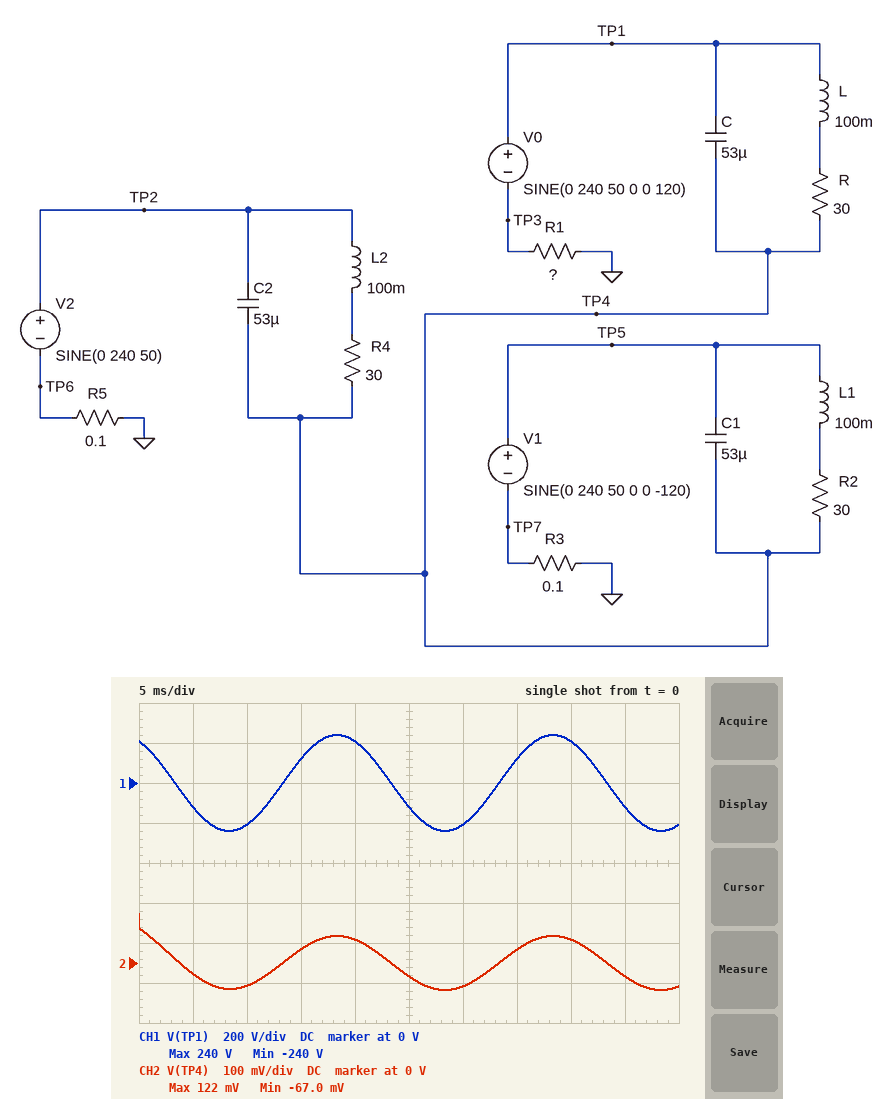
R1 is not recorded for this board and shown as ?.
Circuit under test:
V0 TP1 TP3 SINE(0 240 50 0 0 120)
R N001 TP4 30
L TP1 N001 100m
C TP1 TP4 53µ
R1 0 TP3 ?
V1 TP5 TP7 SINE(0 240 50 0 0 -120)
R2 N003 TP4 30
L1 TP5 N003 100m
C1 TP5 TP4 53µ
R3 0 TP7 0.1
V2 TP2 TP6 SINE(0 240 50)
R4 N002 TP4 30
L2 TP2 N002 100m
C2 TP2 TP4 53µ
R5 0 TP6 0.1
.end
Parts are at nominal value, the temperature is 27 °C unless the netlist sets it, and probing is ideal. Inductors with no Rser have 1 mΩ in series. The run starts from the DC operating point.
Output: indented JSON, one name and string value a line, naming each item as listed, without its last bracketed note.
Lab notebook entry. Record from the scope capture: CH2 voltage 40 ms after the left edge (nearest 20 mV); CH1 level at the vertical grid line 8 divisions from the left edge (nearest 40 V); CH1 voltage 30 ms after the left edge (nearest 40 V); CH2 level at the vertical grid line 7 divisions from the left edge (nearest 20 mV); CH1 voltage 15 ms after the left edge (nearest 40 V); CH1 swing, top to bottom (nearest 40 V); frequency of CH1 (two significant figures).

{
  "CH2 voltage 40 ms after the left edge": "60 mV",
  "CH1 level at the vertical grid line 8 divisions from the left edge": "200 V",
  "CH1 voltage 30 ms after the left edge": "-200 V",
  "CH2 level at the vertical grid line 7 divisions from the left edge": "40 mV",
  "CH1 voltage 15 ms after the left edge": "120 V",
  "CH1 swing, top to bottom": "480 V",
  "frequency of CH1": "50 Hz"
}
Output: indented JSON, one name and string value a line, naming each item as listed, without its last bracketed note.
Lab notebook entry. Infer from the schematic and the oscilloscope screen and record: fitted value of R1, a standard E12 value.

{
  "fitted value of R1, a standard E12 value": "0.047 Ω"
}
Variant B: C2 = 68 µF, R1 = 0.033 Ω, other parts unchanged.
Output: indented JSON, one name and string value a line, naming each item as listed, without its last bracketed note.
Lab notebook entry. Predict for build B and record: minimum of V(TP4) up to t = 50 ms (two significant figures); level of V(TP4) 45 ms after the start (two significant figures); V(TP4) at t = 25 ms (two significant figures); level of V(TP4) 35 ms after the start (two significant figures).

{
  "minimum of V(TP4) up to t = 50 ms": "-24 V",
  "level of V(TP4) 45 ms after the start": "2.3 V",
  "V(TP4) at t = 25 ms": "2.8 V",
  "level of V(TP4) 35 ms after the start": "-2.3 V"
}
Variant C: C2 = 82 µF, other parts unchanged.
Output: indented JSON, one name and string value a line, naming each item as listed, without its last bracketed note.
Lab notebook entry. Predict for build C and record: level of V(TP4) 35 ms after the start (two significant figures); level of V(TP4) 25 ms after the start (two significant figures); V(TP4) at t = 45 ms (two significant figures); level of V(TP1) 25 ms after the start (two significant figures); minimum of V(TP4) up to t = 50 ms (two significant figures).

{
  "level of V(TP4) 35 ms after the start": "-8.6 V",
  "level of V(TP4) 25 ms after the start": "9.5 V",
  "V(TP4) at t = 45 ms": "8.5 V",
  "level of V(TP1) 25 ms after the start": "-120 V",
  "minimum of V(TP4) up to t = 50 ms": "-45 V"
}
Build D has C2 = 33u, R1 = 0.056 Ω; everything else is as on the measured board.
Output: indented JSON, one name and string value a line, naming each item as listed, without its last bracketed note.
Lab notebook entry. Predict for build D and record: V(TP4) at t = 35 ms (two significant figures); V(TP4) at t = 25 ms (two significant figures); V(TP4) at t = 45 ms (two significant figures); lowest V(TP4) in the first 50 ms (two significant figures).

{
  "V(TP4) at t = 35 ms": "-4.2 V",
  "V(TP4) at t = 25 ms": "4.5 V",
  "V(TP4) at t = 45 ms": "4.1 V",
  "lowest V(TP4) in the first 50 ms": "-33 V"
}
